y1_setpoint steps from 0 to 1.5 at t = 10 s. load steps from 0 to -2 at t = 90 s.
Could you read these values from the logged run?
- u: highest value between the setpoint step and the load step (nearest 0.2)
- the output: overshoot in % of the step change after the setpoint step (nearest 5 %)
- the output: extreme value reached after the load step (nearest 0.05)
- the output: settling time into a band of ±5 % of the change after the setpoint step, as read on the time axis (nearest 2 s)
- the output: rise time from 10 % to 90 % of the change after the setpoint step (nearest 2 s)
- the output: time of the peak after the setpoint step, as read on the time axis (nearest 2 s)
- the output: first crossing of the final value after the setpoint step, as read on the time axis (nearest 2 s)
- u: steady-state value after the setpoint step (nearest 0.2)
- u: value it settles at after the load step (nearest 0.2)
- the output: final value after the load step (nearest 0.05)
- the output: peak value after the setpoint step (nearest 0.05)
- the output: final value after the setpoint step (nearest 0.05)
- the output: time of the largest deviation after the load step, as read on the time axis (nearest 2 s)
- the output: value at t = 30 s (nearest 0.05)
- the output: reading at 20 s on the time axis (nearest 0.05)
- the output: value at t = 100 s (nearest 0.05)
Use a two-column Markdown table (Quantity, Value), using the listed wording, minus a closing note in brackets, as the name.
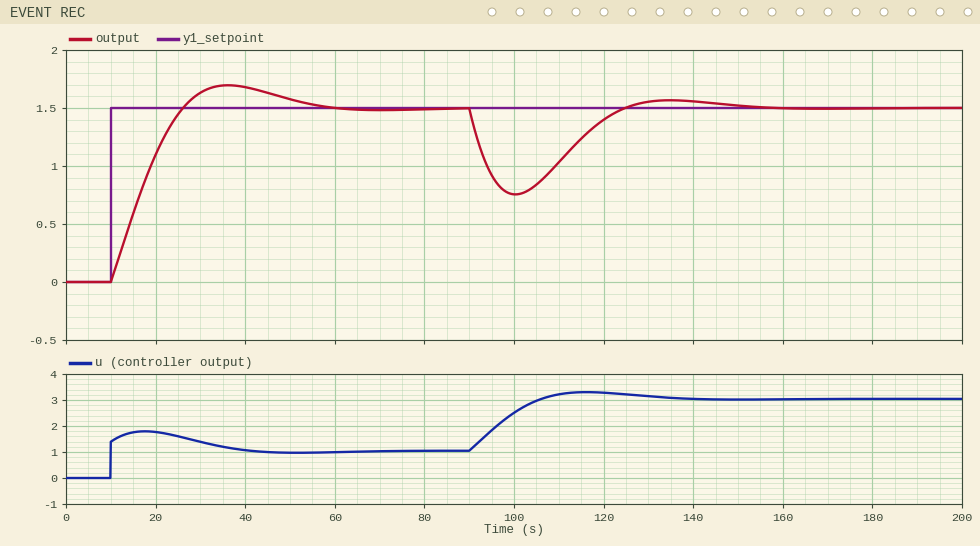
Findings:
| Quantity | Value |
|---|---|
| u: highest value between the setpoint step and the load step | 1.8 |
| the output: overshoot in % of the step change after the setpoint step | 15 % |
| the output: extreme value reached after the load step | 0.75 |
| the output: settling time into a band of ±5 % of the change after the setpoint step, as read on the time axis | 50 s |
| the output: rise time from 10 % to 90 % of the change after the setpoint step | 12 s |
| the output: time of the peak after the setpoint step, as read on the time axis | 36 s |
| the output: first crossing of the final value after the setpoint step, as read on the time axis | 26 s |
| u: steady-state value after the setpoint step | 1.0 |
| u: value it settles at after the load step | 3.0 |
| the output: final value after the load step | 1.50 |
| the output: peak value after the setpoint step | 1.70 |
| the output: final value after the setpoint step | 1.50 |
| the output: time of the largest deviation after the load step, as read on the time axis | 100 s |
| the output: value at t = 30 s | 1.65 |
| the output: reading at 20 s on the time axis | 1.10 |
| the output: value at t = 100 s | 0.75 |
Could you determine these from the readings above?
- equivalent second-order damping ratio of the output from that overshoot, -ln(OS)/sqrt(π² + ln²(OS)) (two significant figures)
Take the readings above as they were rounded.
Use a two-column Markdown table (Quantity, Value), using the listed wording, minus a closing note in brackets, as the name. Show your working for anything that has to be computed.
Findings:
| Quantity | Value |
|---|---|
| equivalent second-order damping ratio of the output from that overshoot, -ln(OS)/sqrt(π² + ln²(OS)) | ln(0.15) = -1.897; 1.897 / sqrt(9.870 + 3.599) = 0.52 |
